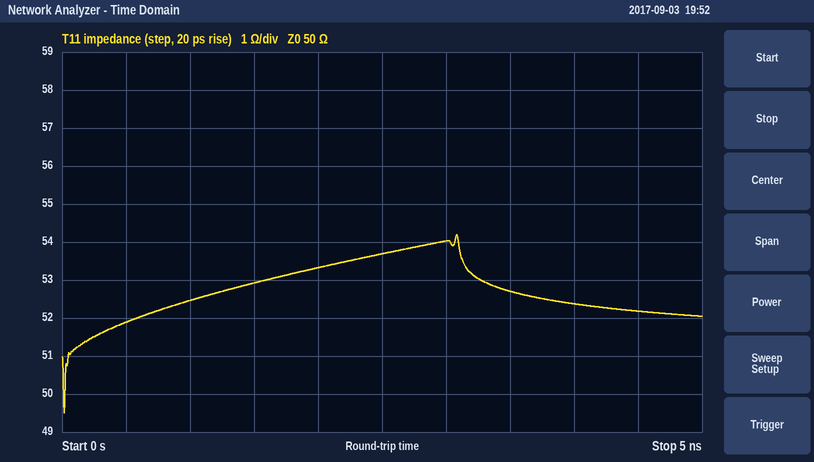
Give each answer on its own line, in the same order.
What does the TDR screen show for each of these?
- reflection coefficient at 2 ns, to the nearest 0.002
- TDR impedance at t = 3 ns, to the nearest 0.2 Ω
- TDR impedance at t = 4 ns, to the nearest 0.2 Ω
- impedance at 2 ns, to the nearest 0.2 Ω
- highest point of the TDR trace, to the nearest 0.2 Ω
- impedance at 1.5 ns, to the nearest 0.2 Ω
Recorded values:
+0.032
54.0 Ω
52.4 Ω
53.4 Ω
54.2 Ω
53.0 Ω
